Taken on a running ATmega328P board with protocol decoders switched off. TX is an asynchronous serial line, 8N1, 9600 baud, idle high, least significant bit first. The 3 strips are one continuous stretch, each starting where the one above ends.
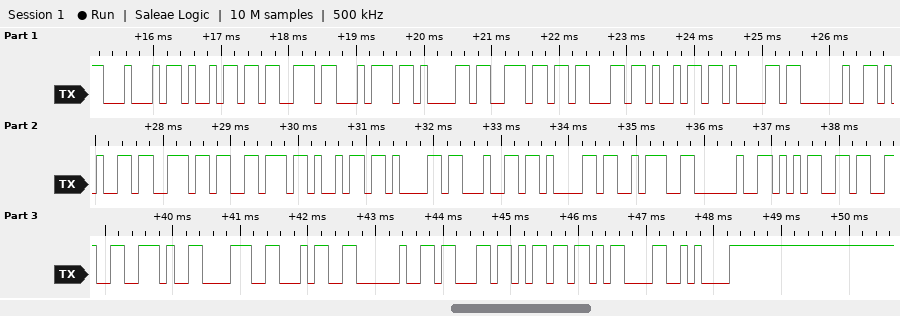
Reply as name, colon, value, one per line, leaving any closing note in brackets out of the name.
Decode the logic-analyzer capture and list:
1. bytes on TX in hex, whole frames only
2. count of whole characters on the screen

bytes on TX in hex, whole frames only: 44 69 73 74 61 6E 63 69 61 20 65 6E 76 69 61 64 61 3A 20 35 33 2E 38 34 20 63 6D 0D 0A
count of whole characters on the screen: 29
